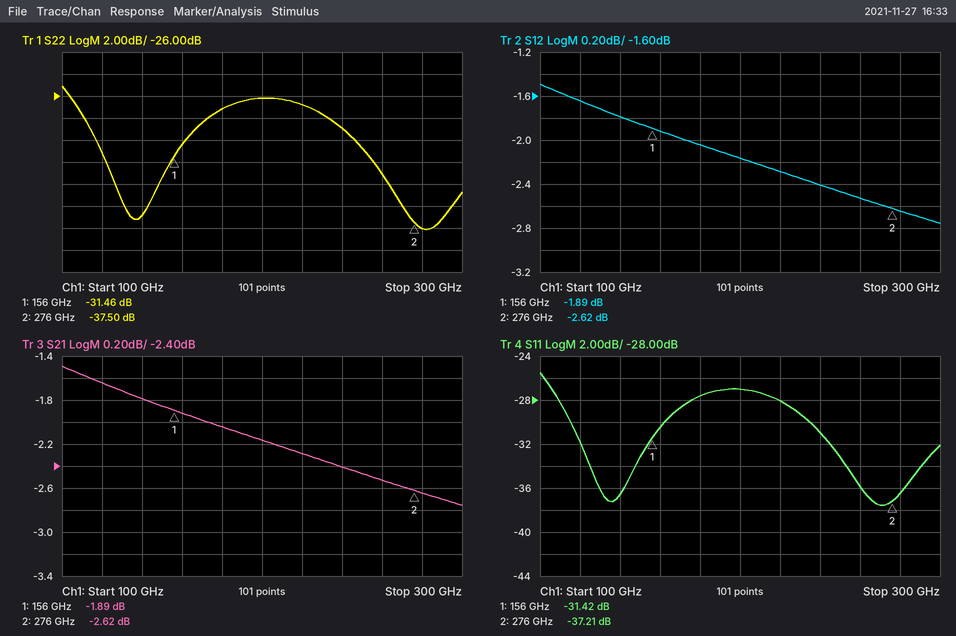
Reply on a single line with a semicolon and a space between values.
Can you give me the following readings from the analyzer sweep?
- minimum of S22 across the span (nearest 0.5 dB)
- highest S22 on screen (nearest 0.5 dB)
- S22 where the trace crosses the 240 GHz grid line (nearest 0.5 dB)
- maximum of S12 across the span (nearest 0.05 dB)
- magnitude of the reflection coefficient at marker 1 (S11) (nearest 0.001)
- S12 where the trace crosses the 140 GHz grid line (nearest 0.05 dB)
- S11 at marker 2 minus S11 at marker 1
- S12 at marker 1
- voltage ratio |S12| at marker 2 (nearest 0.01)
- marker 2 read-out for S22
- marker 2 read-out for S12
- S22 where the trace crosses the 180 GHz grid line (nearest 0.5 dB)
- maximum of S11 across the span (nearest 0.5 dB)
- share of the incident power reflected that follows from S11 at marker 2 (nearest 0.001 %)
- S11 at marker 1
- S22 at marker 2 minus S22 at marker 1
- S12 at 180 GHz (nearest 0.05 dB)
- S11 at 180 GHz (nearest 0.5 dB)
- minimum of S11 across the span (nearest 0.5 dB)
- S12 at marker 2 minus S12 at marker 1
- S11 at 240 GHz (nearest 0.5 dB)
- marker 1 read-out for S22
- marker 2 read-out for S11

-38.0 dB; -25.0 dB; -29.0 dB; -1.50 dB; 0.027; -1.80 dB; -5.79 dB; -1.89 dB; 0.74; -37.50 dB; -2.62 dB; -27.0 dB; -25.5 dB; 0.019 %; -31.42 dB; -6.04 dB; -2.05 dB; -27.5 dB; -37.5 dB; -0.73 dB; -31.0 dB; -31.46 dB; -37.21 dB
